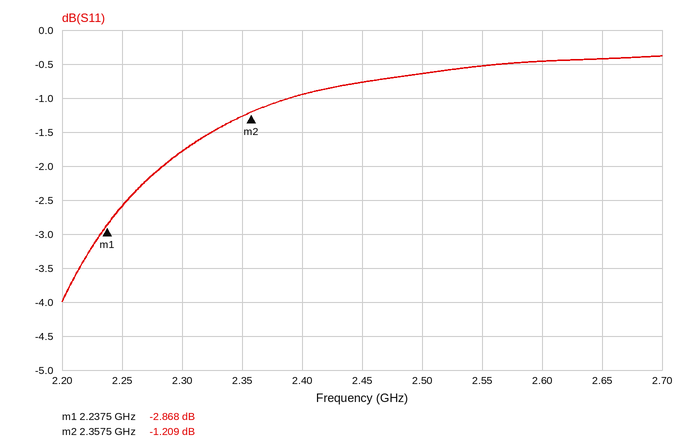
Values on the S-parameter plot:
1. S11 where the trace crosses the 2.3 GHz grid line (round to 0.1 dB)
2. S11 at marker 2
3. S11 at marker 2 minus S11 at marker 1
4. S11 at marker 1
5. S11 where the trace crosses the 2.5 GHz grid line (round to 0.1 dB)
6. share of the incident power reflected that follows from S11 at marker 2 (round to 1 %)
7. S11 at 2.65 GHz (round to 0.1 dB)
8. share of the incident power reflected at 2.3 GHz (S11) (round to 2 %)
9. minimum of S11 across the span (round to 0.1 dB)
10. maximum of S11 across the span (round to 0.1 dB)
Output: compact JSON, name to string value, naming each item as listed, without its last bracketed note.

{"S11 where the trace crosses the 2.3 GHz grid line": "-1.8 dB", "S11 at marker 2": "-1.209 dB", "S11 at marker 2 minus S11 at marker 1": "1.659 dB", "S11 at marker 1": "-2.868 dB", "S11 where the trace crosses the 2.5 GHz grid line": "-0.6 dB", "share of the incident power reflected that follows from S11 at marker 2": "76 %", "S11 at 2.65 GHz": "-0.4 dB", "share of the incident power reflected at 2.3 GHz (S11)": "66 %", "minimum of S11 across the span": "-4.0 dB", "maximum of S11 across the span": "-0.4 dB"}
